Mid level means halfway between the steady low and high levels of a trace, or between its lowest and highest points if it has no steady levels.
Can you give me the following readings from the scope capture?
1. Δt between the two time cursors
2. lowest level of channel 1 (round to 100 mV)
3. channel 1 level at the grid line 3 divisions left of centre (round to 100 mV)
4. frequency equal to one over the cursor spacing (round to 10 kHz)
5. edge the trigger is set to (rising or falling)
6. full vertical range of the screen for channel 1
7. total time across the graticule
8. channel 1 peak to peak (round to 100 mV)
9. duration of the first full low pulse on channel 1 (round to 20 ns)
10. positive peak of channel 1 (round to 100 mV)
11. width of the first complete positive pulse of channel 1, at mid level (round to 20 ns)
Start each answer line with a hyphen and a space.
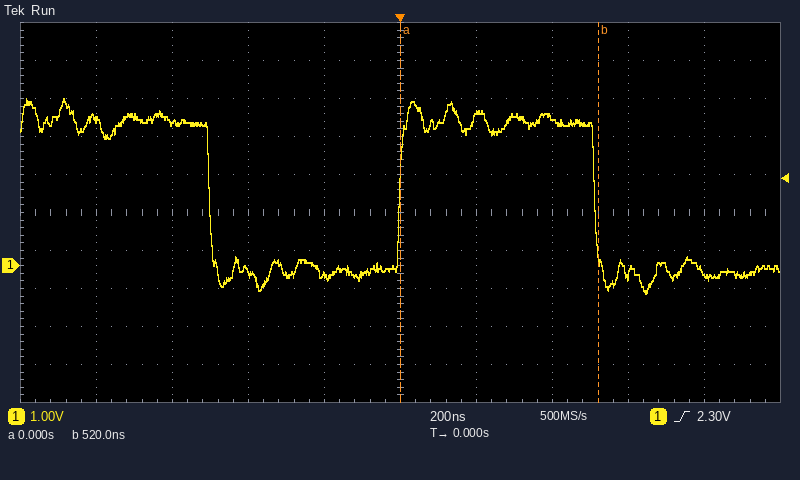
- 520 ns
- -700 mV
- 3.8 V
- 1.92 MHz
- rising
- 10 V
- 2 µs
- 5.1 V
- 500 ns
- 4.4 V
- 520 ns
